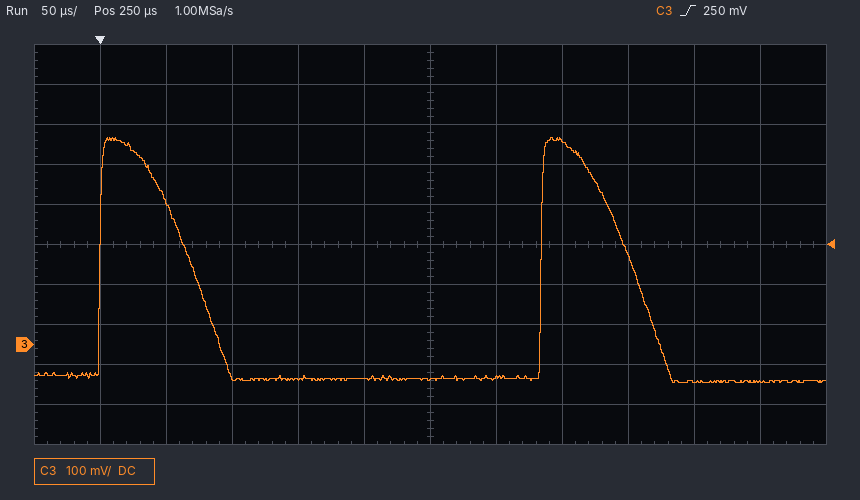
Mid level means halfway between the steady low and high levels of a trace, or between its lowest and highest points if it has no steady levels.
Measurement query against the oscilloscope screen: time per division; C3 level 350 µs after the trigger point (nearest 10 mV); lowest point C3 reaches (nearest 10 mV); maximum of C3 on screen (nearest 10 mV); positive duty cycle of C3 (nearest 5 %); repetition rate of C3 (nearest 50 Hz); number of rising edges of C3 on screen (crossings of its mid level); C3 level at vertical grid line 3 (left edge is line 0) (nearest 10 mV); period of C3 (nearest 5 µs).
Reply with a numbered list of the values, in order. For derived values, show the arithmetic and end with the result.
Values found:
1. 50 µs
2. 510 mV
3. -100 mV
4. 520 mV
5. 20 %
6. 1 / 335 µs ≈ 2.99 kHz, so 3.00 kHz to the nearest 50 Hz
7. 2
8. -80 mV
9. 335 µs
